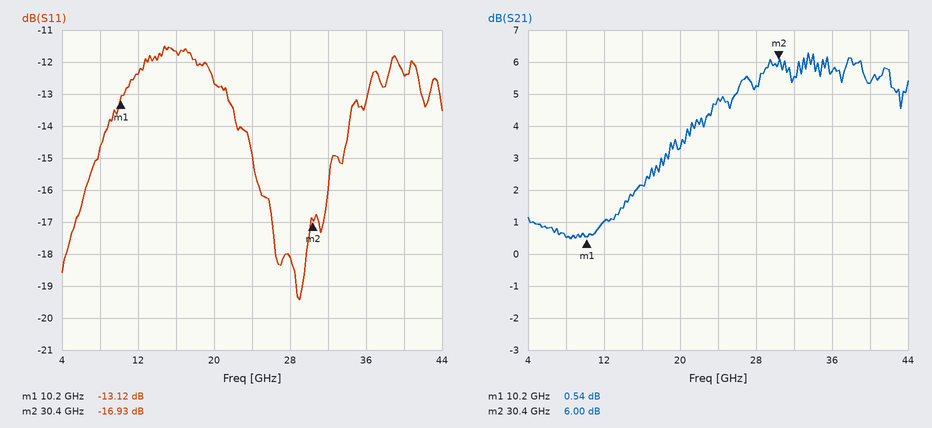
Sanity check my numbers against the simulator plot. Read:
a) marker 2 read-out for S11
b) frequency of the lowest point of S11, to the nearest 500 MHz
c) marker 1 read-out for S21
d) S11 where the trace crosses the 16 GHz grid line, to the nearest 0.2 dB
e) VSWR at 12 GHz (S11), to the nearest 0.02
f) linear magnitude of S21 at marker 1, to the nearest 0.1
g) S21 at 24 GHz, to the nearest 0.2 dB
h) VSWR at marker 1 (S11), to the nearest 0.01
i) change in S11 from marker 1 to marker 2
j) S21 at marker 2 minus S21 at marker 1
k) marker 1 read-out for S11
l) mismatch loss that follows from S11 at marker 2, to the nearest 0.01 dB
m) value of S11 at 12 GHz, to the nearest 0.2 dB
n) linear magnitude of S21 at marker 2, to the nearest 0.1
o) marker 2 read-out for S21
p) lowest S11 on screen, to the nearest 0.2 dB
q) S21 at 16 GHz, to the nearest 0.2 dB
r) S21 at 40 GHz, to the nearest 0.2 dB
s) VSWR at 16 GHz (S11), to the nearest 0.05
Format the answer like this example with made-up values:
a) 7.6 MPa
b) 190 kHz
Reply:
a) -16.93 dB
b) 29.0 GHz
c) 0.54 dB
d) -11.6 dB
e) 1.64
f) 1.1
g) 4.8 dB
h) 1.57
i) -3.81 dB
j) 5.46 dB
k) -13.12 dB
l) 0.09 dB
m) -12.4 dB
n) 2.0
o) 6.00 dB
p) -19.4 dB
q) 2.2 dB
r) 5.4 dB
s) 1.70
